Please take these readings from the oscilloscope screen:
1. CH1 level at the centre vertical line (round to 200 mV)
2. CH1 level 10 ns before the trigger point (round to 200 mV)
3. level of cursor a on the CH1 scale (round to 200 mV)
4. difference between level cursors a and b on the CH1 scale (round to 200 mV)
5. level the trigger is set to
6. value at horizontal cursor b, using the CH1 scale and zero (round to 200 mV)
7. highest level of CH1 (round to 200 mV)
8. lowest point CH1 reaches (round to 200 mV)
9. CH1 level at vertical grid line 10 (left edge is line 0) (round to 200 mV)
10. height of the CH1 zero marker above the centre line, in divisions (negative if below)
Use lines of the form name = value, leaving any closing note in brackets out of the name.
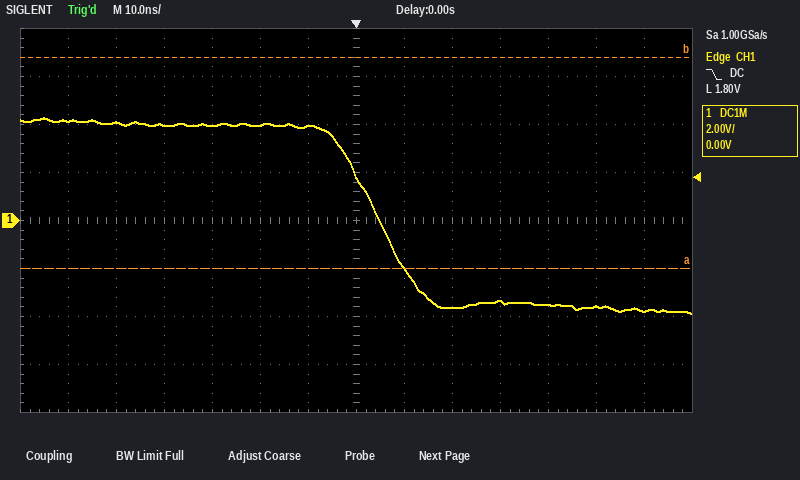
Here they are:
CH1 level at the centre vertical line = 1.8 V
CH1 level 10 ns before the trigger point = 4.0 V
level of cursor a on the CH1 scale = -2.0 V
difference between level cursors a and b on the CH1 scale = 8.8 V
level the trigger is set to = 1.80 V
value at horizontal cursor b, using the CH1 scale and zero = 6.8 V
highest level of CH1 = 4.2 V
lowest point CH1 reaches = -3.8 V
CH1 level at vertical grid line 10 (left edge is line 0) = -3.4 V
height of the CH1 zero marker above the centre line, in divisions = 0.0 div
